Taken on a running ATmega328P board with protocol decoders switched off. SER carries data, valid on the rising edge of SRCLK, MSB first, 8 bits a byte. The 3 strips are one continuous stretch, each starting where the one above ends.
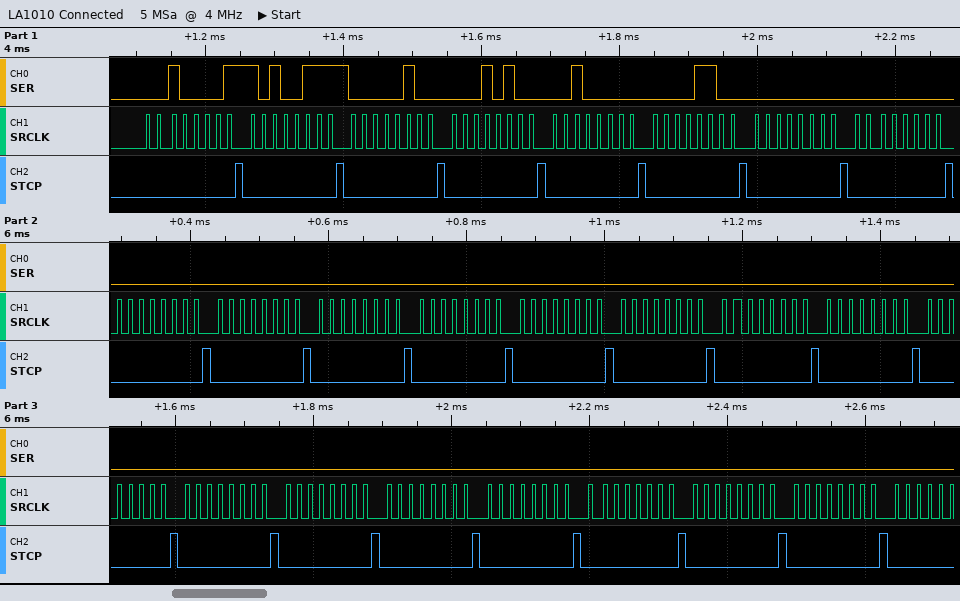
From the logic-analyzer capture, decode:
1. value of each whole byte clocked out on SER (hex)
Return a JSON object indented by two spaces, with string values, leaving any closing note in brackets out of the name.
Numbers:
{
  "value of each whole byte clocked out on SER": "21 A7 04 14 20 0C 00 00 00 00 00 00 00 00 00 00 00 00 00 00 00 00 00 00"
}
